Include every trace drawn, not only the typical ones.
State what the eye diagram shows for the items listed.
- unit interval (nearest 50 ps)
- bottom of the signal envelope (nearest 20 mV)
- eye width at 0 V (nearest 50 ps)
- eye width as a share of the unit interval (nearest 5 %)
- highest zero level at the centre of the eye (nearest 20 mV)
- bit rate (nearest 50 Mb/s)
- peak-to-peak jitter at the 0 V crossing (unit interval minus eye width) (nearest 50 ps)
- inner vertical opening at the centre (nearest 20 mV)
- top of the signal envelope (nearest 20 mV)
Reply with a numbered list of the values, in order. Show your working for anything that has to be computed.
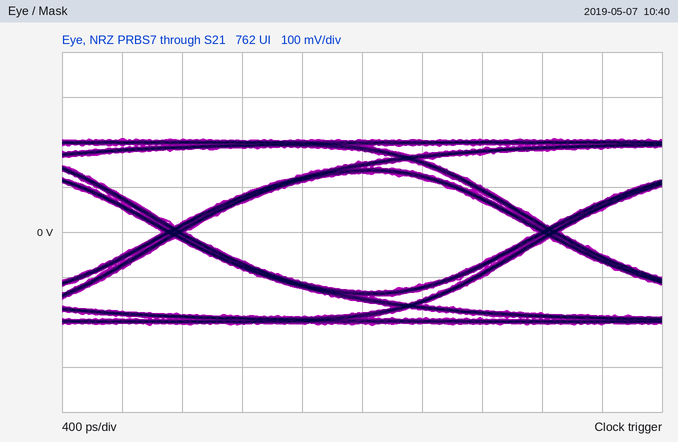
1. 2.50 ns
2. -200 mV
3. 2.35 ns
4. 2.35 ns / 2.50 ns ≈ 94.0 %, so 95 % to the nearest 5 %
5. -140 mV
6. 400 Mb/s
7. 150 ps
8. 260 mV
9. 200 mV
